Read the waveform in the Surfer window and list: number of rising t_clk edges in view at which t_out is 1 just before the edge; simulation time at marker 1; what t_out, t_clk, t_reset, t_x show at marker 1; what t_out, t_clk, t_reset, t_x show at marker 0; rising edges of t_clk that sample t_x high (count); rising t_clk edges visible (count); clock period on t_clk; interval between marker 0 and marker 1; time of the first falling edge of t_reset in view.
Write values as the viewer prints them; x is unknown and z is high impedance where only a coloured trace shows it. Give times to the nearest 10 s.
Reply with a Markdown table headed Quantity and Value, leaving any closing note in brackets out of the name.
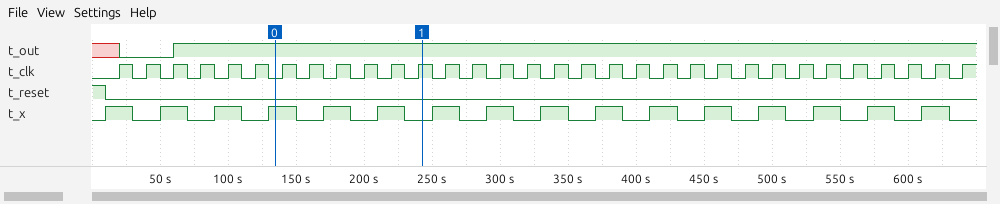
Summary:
| Quantity | Value |
|---|---|
| number of rising t_clk edges in view at which t_out is 1 just before the edge | 29 |
| simulation time at marker 1 | 240 s |
| what t_out, t_clk, t_reset, t_x show at marker 1 | t_out=1, t_clk=1, t_reset=0, t_x=0 |
| what t_out, t_clk, t_reset, t_x show at marker 0 | t_out=1, t_clk=0, t_reset=0, t_x=1 |
| rising edges of t_clk that sample t_x high | 16 |
| rising t_clk edges visible | 32 |
| clock period on t_clk | 20 s |
| interval between marker 0 and marker 1 | 110 s |
| time of the first falling edge of t_reset in view | 10 s |
